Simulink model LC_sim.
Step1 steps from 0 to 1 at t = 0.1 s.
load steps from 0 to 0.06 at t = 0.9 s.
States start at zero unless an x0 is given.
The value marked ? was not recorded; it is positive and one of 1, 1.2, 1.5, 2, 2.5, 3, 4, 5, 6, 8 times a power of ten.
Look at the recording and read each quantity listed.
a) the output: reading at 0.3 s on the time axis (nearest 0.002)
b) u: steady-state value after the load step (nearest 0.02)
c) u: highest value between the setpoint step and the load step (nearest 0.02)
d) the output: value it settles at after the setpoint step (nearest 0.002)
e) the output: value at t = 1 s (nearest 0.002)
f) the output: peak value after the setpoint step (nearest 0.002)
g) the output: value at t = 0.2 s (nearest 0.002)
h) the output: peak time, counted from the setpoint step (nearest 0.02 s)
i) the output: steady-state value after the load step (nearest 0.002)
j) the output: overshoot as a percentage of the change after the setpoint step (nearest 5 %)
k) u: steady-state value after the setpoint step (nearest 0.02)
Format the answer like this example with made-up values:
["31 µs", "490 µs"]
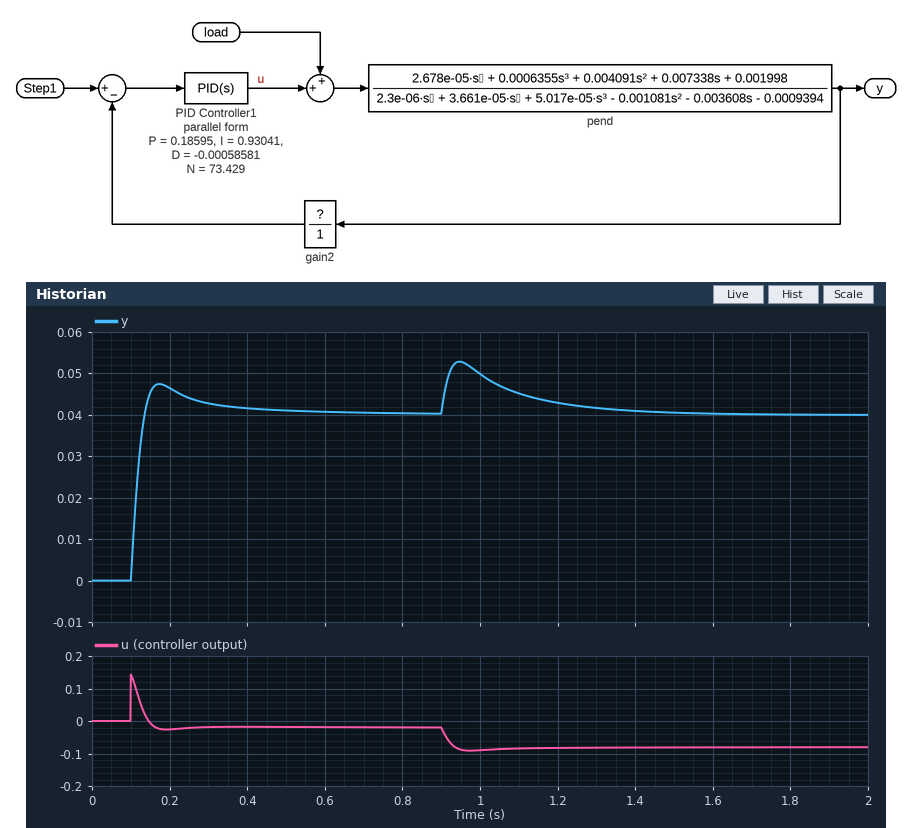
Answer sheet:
["0.042", "-0.08", "0.14", "0.040", "0.050", "0.048", "0.046", "0.08 s", "0.040", "20 %", "-0.02"]
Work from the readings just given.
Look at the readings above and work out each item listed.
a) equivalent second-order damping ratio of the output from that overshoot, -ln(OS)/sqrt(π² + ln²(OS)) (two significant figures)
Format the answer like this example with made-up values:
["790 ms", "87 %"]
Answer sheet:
["0.46"]
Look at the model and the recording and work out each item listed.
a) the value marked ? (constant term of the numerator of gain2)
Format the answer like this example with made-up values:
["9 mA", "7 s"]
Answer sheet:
["25"]
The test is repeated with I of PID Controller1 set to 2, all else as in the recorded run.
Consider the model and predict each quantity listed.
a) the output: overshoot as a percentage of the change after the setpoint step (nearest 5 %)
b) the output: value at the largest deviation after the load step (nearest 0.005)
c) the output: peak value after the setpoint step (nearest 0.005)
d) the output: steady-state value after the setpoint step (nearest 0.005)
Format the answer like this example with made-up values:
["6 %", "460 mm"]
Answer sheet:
["25 %", "0.050", "0.050", "0.040"]
